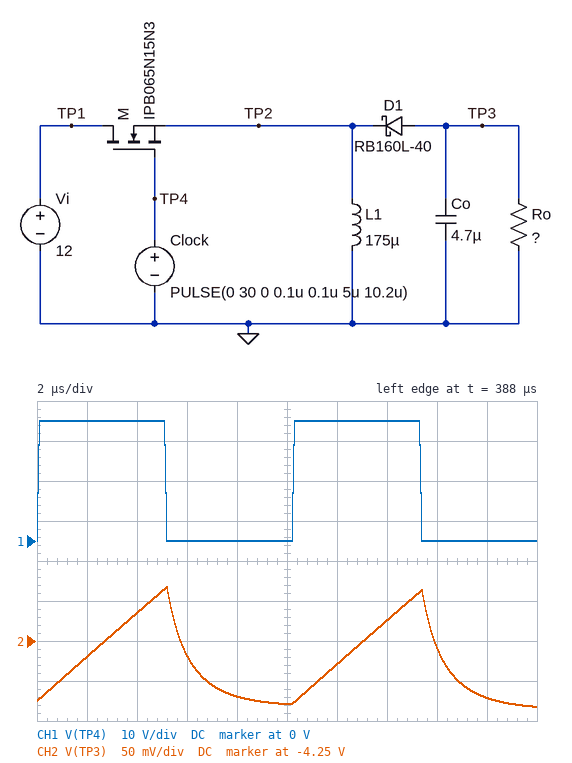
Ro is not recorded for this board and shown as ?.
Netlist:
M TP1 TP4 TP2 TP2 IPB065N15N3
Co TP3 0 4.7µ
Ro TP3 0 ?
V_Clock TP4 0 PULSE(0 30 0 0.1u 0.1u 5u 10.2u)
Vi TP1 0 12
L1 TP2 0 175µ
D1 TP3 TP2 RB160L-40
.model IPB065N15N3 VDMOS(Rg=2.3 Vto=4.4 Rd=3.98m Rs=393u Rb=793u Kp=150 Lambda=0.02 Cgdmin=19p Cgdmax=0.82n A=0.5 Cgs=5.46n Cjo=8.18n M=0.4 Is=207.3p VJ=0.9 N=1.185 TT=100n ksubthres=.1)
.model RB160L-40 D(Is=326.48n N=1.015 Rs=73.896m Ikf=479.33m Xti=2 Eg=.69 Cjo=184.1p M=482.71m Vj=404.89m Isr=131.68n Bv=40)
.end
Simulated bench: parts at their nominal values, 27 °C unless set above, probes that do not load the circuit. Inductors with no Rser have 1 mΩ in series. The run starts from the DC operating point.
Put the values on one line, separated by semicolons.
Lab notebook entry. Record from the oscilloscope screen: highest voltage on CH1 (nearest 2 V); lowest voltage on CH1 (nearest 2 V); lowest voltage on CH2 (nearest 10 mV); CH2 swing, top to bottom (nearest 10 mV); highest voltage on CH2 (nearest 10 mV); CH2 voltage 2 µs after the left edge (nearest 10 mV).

30 V; 0 V; -4.33 V; 150 mV; -4.18 V; -4.27 V
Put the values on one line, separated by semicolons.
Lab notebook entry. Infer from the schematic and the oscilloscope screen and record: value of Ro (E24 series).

33 Ω
